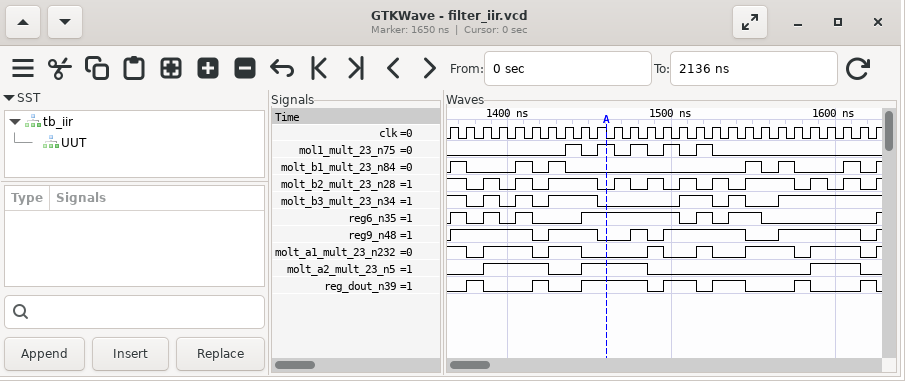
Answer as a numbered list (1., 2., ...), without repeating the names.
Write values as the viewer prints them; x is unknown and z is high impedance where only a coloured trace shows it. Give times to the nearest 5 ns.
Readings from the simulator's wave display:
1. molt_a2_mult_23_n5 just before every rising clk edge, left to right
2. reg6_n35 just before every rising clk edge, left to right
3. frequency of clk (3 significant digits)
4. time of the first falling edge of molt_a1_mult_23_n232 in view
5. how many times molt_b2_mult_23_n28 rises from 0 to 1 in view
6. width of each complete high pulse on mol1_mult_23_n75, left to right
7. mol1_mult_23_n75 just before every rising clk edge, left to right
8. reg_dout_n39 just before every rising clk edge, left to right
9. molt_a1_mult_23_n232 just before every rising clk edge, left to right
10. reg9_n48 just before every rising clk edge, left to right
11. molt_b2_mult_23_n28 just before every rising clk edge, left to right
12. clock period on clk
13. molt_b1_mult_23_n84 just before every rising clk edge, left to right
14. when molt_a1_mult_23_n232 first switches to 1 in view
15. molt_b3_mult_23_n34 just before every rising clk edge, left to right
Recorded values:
1. 0 0 0 1 1 1 1 0 0 1 1 1 1 0 0 0 0 0 0 0 0 0 0 1 1 1 0
2. 0 1 0 1 0 1 0 0 0 1 1 1 1 1 1 0 1 0 1 1 0 0 0 0 0 0 0
3. 100 MHz
4. 1375 ns
5. 11
6. 10 ns, 10 ns, 10 ns, 10 ns, 10 ns
7. 0 0 0 0 0 0 0 0 1 0 1 0 1 0 1 0 1 0 0 0 0 0 0 0 0 0 0
8. 0 0 1 0 0 0 1 0 0 1 1 1 1 0 1 1 0 1 1 0 0 0 1 0 0 0 1
9. 1 1 0 1 1 1 0 1 1 0 0 0 0 1 0 0 1 0 0 1 1 1 0 1 1 1 0
10. 0 1 1 1 1 1 0 1 1 1 0 0 1 0 1 1 1 1 1 0 0 1 1 1 1 1 0
11. 1 1 0 1 0 1 0 1 1 1 0 1 0 1 0 1 0 1 0 1 1 1 0 1 0 1 0
12. 10 ns
13. 0 1 0 0 0 1 0 1 0 0 0 0 0 0 0 0 0 0 0 1 0 1 0 0 0 1 0
14. 1385 ns
15. 1 1 0 1 0 1 0 1 1 1 0 0 0 0 0 1 1 0 1 0 0 1 1 1 1 1 1
